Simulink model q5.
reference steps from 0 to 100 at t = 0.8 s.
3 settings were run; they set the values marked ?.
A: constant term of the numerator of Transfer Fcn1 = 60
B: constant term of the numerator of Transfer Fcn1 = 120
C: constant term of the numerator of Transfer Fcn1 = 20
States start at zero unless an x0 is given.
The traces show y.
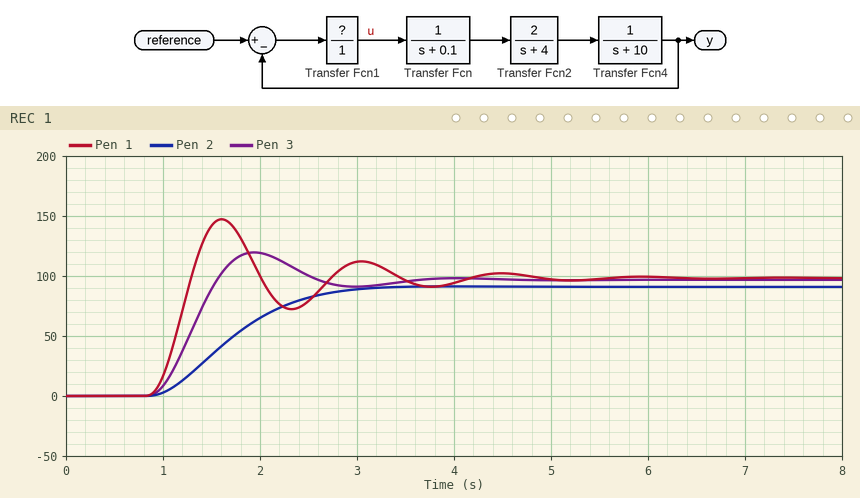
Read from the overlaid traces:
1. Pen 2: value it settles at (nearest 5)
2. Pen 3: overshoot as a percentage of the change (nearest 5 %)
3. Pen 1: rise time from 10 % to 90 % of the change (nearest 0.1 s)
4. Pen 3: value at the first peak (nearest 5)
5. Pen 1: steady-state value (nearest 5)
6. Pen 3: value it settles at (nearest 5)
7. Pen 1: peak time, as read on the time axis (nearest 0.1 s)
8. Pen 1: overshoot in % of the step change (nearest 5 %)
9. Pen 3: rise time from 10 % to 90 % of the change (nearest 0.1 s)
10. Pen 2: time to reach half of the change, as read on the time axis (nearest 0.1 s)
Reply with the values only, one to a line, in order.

90
25 %
0.3 s
120
100
95
1.6 s
50 %
0.5 s
1.7 s
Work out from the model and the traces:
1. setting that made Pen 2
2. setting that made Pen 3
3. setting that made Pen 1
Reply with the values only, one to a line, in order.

C
A
B
